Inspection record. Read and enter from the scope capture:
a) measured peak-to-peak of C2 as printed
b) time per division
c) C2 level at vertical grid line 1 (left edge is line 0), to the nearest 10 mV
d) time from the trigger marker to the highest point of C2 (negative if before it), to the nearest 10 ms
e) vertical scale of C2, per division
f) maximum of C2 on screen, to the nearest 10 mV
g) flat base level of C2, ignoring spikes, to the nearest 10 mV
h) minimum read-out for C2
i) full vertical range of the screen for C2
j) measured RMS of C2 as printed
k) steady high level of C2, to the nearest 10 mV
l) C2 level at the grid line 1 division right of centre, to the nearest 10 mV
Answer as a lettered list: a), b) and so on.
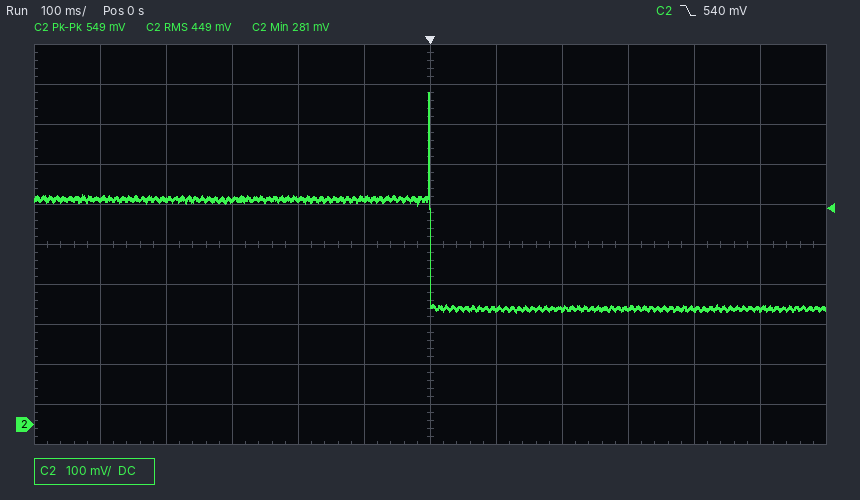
a) 549 mV
b) 100 ms
c) 560 mV
d) 0 ms
e) 100 mV
f) 830 mV
g) 290 mV
h) 281 mV
i) 1 V
j) 449 mV
k) 560 mV
l) 290 mV
